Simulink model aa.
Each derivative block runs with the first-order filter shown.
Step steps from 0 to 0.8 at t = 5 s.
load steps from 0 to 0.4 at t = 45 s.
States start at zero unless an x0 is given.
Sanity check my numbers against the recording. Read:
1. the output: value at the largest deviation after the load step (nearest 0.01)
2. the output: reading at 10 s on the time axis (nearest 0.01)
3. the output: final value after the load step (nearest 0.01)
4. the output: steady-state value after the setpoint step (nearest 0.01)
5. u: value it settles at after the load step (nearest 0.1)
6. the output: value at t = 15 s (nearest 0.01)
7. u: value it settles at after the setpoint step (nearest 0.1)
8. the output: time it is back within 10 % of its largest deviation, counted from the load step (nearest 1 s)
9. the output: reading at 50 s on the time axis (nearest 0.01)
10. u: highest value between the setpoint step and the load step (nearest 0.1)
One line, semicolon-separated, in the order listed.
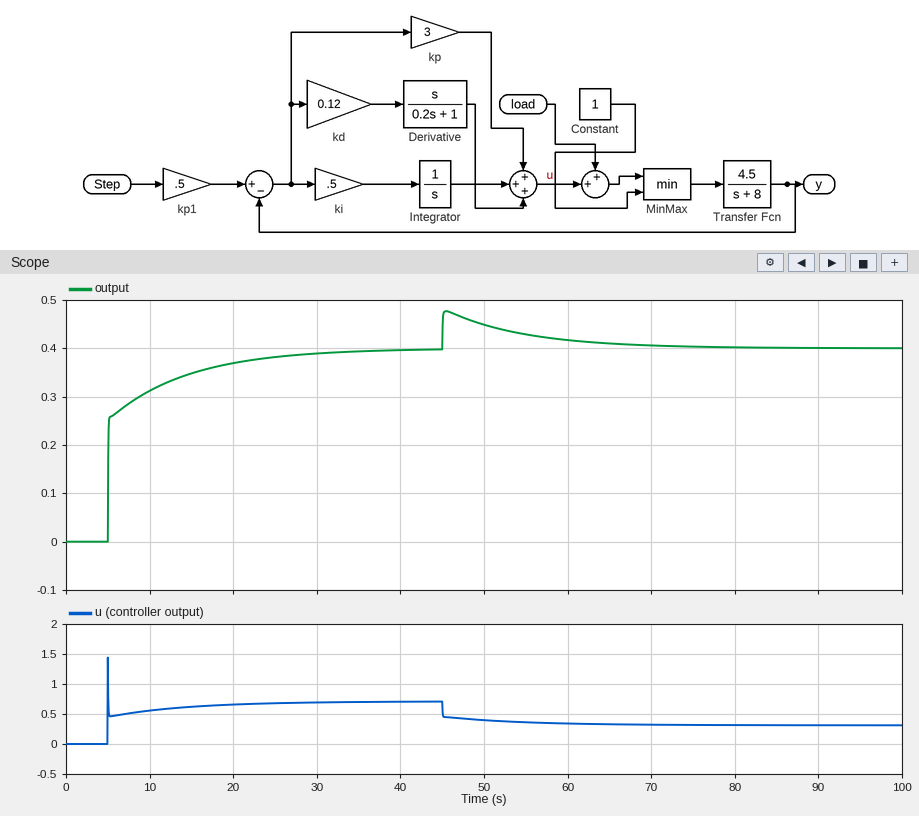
0.48; 0.31; 0.40; 0.40; 0.3; 0.35; 0.7; 22 s; 0.45; 1.4
